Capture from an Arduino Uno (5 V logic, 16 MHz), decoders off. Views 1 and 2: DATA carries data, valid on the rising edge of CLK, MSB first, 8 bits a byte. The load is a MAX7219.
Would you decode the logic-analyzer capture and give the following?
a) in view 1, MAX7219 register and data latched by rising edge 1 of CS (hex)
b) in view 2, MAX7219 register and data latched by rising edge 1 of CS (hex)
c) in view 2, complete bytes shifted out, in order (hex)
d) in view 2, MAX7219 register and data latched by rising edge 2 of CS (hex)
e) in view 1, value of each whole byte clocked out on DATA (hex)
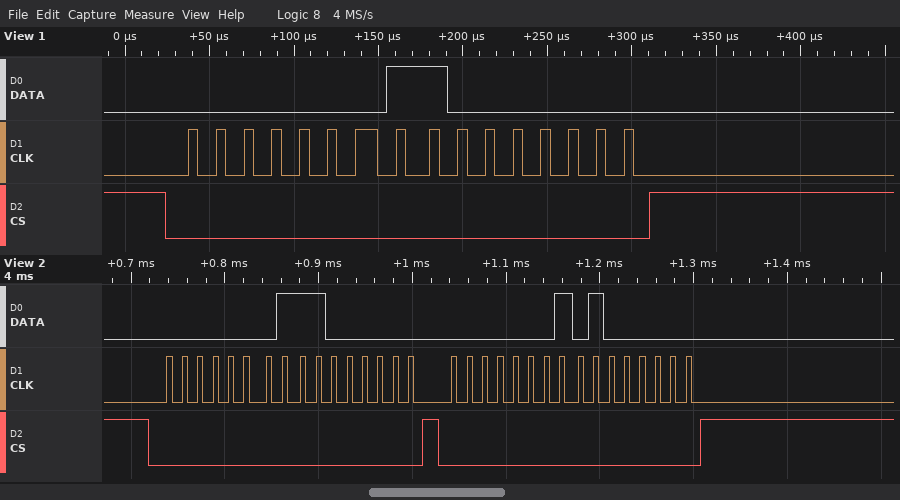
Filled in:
register 0x1, data 0x80
register 0x1, data 0xC0
01 C0 01 40
register 0x1, data 0x40
01 80
